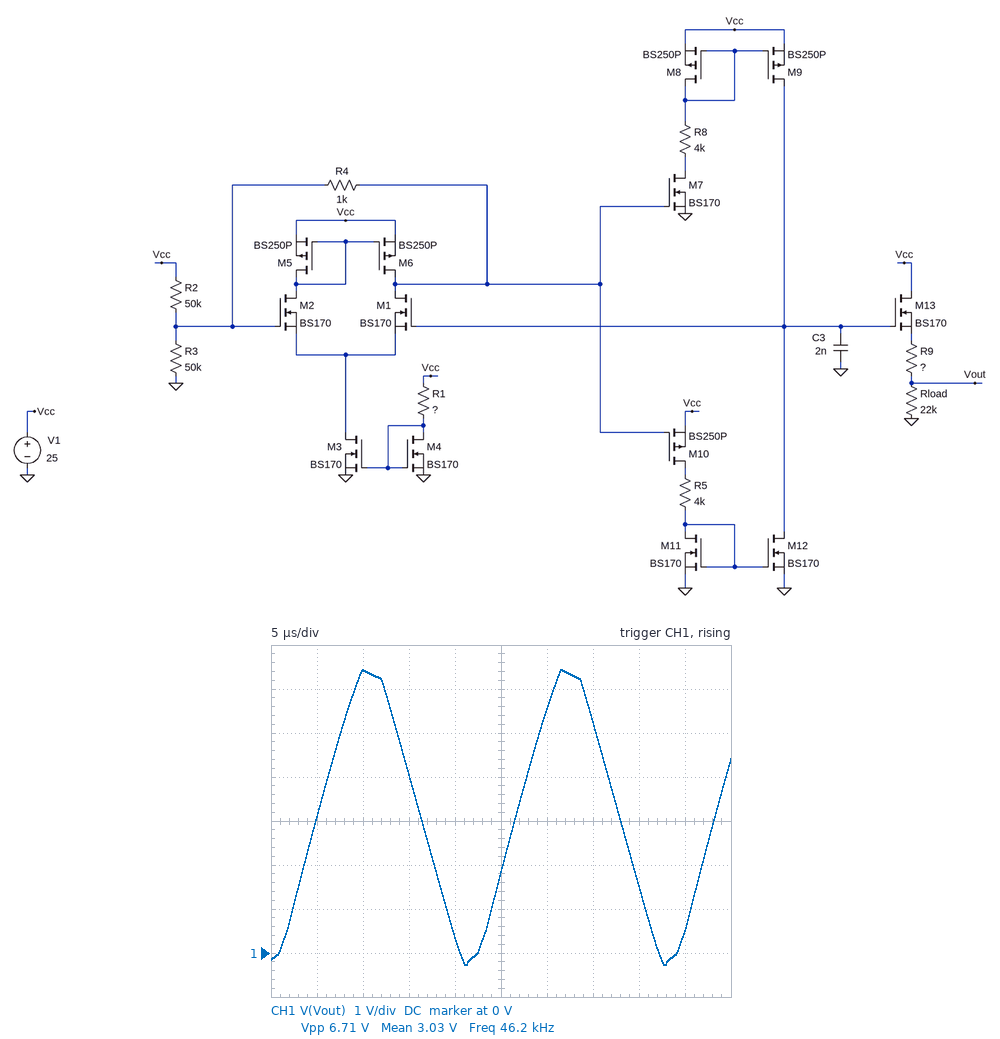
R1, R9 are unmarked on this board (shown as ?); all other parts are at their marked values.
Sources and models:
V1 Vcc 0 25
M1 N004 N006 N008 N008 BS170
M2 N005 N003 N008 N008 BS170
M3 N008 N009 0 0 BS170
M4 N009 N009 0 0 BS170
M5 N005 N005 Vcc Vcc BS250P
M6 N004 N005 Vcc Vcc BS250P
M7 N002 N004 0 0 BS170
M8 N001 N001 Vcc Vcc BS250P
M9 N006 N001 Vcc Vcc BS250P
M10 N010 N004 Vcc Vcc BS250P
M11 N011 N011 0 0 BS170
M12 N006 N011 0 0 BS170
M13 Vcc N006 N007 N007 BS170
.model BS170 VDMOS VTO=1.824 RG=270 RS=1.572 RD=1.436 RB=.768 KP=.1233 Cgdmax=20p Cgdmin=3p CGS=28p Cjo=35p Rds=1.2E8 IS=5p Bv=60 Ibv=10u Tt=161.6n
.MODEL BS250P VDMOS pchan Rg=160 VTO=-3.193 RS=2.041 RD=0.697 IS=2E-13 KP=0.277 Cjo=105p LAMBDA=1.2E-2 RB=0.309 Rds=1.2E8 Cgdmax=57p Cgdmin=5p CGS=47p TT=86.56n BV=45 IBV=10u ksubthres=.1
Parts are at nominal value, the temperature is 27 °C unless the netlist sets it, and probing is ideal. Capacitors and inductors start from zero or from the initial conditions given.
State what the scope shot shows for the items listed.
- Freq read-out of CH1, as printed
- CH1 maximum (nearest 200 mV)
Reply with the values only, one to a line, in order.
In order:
46.2 kHz
6.4 V
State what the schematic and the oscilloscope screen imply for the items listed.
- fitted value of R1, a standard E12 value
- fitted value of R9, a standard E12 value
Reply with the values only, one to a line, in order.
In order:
6.8 kΩ
56 kΩ
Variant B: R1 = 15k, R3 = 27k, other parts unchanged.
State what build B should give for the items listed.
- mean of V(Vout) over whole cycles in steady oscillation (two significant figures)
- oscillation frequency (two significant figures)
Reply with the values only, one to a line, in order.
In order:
3.3 V
40 kHz
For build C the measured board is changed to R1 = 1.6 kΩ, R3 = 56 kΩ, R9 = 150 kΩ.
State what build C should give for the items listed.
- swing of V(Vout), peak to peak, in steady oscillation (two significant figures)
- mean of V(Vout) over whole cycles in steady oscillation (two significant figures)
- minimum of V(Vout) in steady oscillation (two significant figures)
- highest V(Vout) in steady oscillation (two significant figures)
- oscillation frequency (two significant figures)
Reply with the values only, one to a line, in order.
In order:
3.0 V
1.4 V
-120 mV
2.9 V
52 kHz
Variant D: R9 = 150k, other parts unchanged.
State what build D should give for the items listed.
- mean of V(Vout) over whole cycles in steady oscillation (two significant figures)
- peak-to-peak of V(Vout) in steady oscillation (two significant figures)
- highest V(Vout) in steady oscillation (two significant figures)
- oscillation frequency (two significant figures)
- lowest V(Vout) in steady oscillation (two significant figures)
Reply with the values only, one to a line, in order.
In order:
1.5 V
3.0 V
2.9 V
46 kHz
-120 mV
